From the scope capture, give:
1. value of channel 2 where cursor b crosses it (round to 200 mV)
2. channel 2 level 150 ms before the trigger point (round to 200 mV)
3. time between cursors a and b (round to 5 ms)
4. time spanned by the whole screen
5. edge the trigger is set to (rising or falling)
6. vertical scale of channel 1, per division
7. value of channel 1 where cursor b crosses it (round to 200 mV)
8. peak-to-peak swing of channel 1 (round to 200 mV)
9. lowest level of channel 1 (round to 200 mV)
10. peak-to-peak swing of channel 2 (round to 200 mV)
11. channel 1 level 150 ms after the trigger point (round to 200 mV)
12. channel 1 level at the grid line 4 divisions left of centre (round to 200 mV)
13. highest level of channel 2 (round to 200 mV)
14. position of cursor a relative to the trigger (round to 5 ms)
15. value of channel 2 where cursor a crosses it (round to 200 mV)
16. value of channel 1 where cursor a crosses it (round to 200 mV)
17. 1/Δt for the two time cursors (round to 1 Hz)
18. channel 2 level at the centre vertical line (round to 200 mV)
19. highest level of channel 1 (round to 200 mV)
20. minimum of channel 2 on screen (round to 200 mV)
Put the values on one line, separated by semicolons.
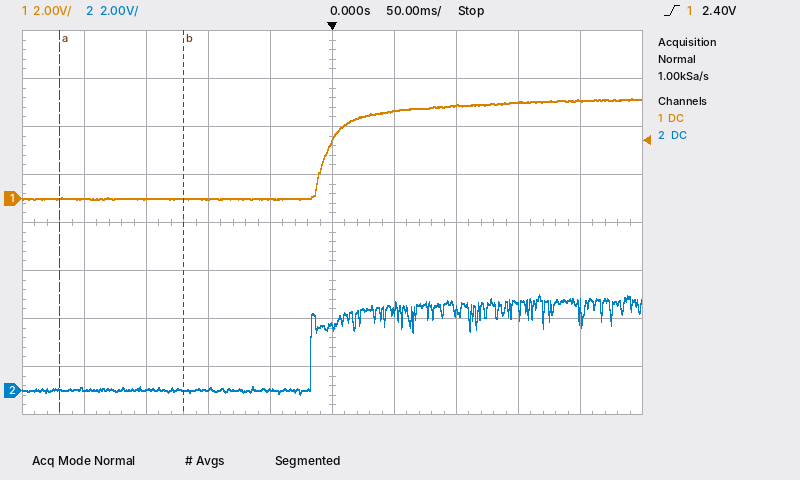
0.0 V; 0.0 V; 100 ms; 500 ms; rising; 2 V; 0.0 V; 4.2 V; 0.0 V; 4.2 V; 4.0 V; 0.0 V; 4.0 V; -220 ms; 0.0 V; 0.0 V; 10 Hz; 2.6 V; 4.2 V; -200 mV
